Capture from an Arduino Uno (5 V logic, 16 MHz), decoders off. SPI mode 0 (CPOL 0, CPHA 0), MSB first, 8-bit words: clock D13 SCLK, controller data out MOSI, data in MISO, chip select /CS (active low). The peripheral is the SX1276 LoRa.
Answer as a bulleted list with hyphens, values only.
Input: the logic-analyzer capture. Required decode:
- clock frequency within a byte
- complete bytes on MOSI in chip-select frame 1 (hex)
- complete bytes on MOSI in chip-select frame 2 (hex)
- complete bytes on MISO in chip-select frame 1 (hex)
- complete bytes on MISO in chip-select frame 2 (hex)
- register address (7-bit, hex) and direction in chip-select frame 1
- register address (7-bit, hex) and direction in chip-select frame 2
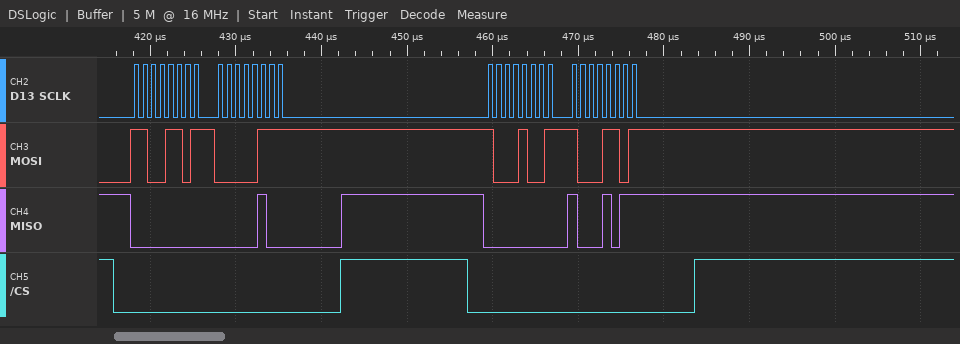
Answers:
- 1 MHz
- CD 07
- 89 8D
- 00 04
- 00 8B
- 0x4D write
- 0x09 write
